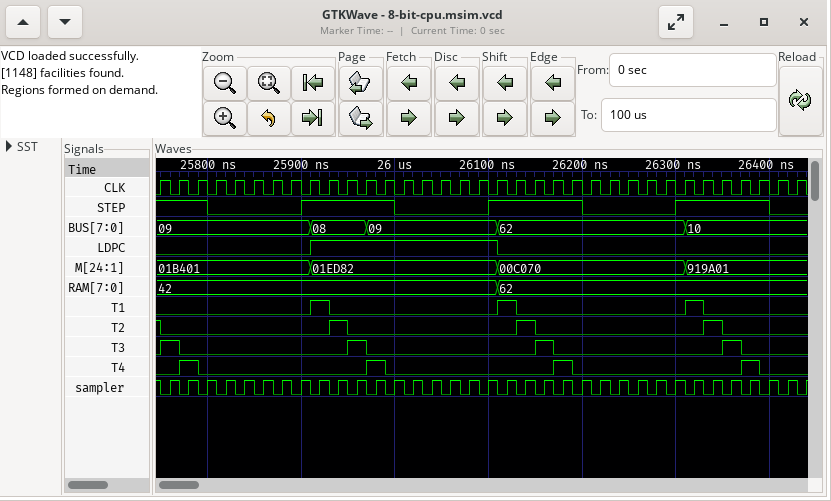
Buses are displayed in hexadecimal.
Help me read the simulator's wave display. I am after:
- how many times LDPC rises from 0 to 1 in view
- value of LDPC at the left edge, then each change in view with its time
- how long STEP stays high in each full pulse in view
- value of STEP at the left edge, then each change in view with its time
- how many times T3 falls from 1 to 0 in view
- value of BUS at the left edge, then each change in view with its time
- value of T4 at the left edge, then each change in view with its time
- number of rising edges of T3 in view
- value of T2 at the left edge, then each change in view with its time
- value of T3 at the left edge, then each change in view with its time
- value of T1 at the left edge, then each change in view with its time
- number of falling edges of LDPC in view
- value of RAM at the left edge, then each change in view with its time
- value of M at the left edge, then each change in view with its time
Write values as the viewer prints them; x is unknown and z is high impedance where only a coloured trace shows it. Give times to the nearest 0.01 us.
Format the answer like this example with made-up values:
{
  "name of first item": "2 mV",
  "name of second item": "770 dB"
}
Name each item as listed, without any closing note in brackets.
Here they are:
{
  "how many times LDPC rises from 0 to 1 in view": "1",
  "value of LDPC at the left edge, then each change in view with its time": "0, 1 at 25.91 us, 0 at 26.11 us",
  "how long STEP stays high in each full pulse in view": "0.1 us, 0.1 us, 0.1 us",
  "value of STEP at the left edge, then each change in view with its time": "1, 0 at 25.8 us, 1 at 25.9 us, 0 at 26 us, 1 at 26.1 us, 0 at 26.2 us, 1 at 26.3 us, 0 at 26.4 us",
  "how many times T3 falls from 1 to 0 in view": "4",
  "value of BUS at the left edge, then each change in view with its time": "09, 08 at 25.91 us, 09 at 25.97 us, 62 at 26.11 us, 10 at 26.31 us",
  "value of T4 at the left edge, then each change in view with its time": "0, 1 at 25.77 us, 0 at 25.79 us, 1 at 25.97 us, 0 at 25.99 us, 1 at 26.17 us, 0 at 26.19 us, 1 at 26.37 us, 0 at 26.39 us",
  "number of rising edges of T3 in view": "4",
  "value of T2 at the left edge, then each change in view with its time": "1, 0 at 25.75 us, 1 at 25.93 us, 0 at 25.95 us, 1 at 26.13 us, 0 at 26.15 us, 1 at 26.33 us, 0 at 26.35 us",
  "value of T3 at the left edge, then each change in view with its time": "0, 1 at 25.75 us, 0 at 25.77 us, 1 at 25.95 us, 0 at 25.97 us, 1 at 26.15 us, 0 at 26.17 us, 1 at 26.35 us, 0 at 26.37 us",
  "value of T1 at the left edge, then each change in view with its time": "0, 1 at 25.91 us, 0 at 25.93 us, 1 at 26.11 us, 0 at 26.13 us, 1 at 26.31 us, 0 at 26.33 us",
  "number of falling edges of LDPC in view": "1",
  "value of RAM at the left edge, then each change in view with its time": "42, 62 at 26.11 us",
  "value of M at the left edge, then each change in view with its time": "01B401, 01ED82 at 25.91 us, 00C070 at 26.11 us, 919A01 at 26.31 us"
}
